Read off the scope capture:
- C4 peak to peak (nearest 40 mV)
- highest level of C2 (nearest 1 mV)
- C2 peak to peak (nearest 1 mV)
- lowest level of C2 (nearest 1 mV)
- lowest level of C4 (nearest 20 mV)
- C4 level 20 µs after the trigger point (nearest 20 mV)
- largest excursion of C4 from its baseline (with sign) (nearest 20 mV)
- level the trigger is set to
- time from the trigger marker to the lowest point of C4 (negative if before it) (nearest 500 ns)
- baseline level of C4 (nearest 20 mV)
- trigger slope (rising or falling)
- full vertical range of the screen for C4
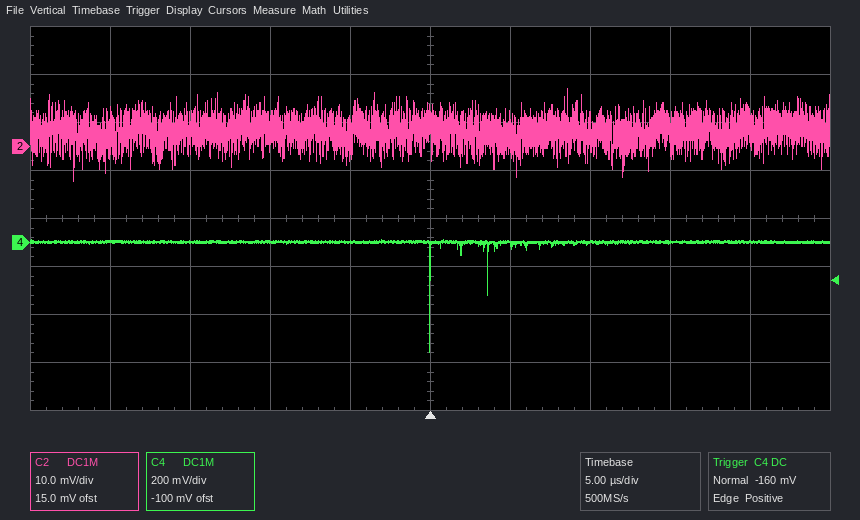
480 mV
12 mV
19 mV
-7 mV
-460 mV
0 mV
-460 mV
-160 mV
0.0 µs
0 mV
rising
1.6 V
